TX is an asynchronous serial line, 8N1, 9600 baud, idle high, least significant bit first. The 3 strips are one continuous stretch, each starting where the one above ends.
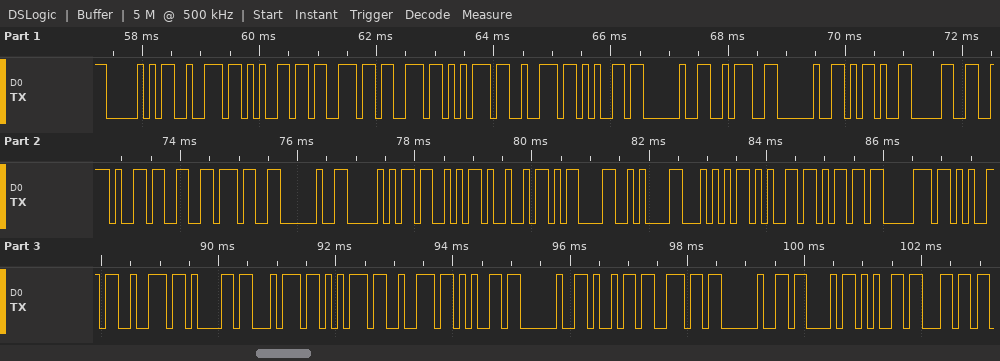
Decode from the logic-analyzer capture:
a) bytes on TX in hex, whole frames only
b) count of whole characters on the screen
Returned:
50 72 65 73 73 75 72 65 20 3A 20 2D 30 2E 33 37 20 50 53 49 0D 0A 54 65 6D 70 65 72 61 74 75 72 65 20 69 6E 20 43 65 6C
40
